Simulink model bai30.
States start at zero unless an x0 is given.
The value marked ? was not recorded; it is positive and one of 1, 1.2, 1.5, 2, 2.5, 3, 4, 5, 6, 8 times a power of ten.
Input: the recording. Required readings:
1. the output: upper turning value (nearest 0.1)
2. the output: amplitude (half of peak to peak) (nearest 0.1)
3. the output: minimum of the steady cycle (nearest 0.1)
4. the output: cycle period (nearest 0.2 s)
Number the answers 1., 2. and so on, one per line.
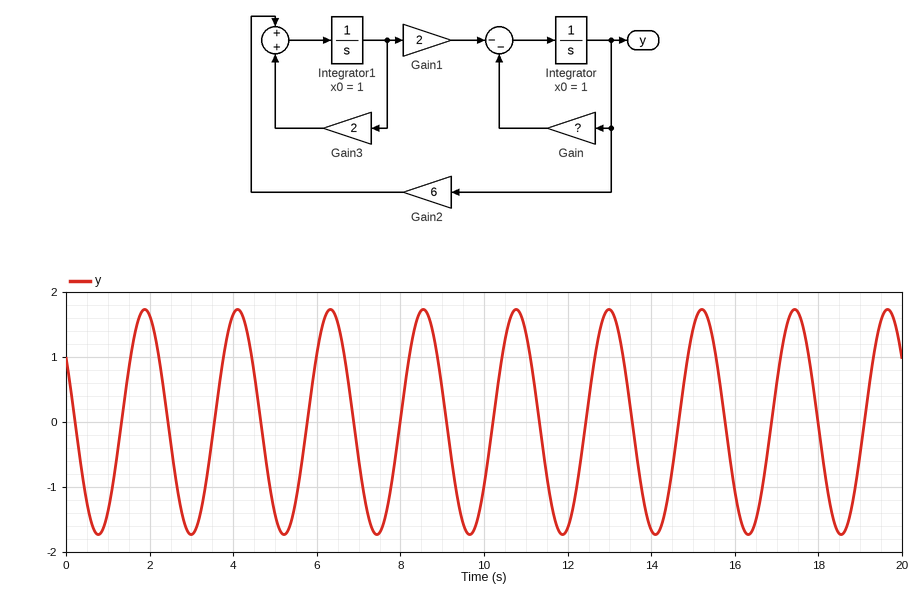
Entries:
1. 1.7
2. 1.7
3. -1.7
4. 2.2 s
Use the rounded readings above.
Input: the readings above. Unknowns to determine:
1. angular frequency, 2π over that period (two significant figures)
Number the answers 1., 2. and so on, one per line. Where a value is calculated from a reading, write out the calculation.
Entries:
1. 2π / 2.2 = 2.9 rad/s
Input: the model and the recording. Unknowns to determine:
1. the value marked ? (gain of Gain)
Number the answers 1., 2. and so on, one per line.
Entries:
1. 2
